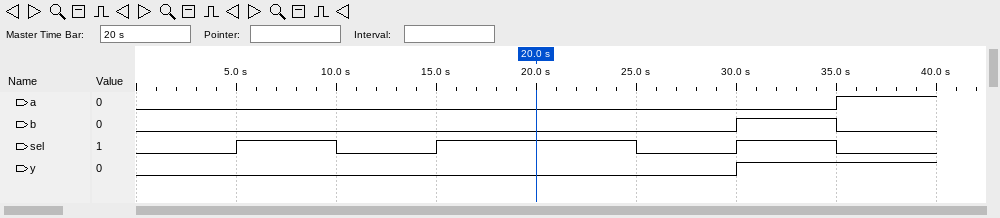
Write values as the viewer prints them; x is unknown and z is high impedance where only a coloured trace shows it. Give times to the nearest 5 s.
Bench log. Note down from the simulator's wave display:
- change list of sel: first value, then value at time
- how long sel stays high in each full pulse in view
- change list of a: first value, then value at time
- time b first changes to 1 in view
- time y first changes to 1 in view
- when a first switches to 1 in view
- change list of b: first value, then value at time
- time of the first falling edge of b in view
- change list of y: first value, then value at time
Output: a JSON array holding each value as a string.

["0, 1 at 5 s, 0 at 10 s, 1 at 15 s, 0 at 25 s, 1 at 30 s, 0 at 35 s", "5 s, 10 s, 5 s", "0, 1 at 35 s", "30 s", "30 s", "35 s", "0, 1 at 30 s, 0 at 35 s", "35 s", "0, 1 at 30 s"]
